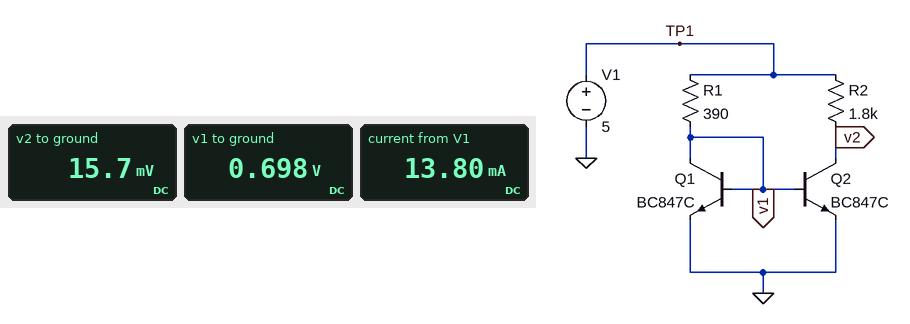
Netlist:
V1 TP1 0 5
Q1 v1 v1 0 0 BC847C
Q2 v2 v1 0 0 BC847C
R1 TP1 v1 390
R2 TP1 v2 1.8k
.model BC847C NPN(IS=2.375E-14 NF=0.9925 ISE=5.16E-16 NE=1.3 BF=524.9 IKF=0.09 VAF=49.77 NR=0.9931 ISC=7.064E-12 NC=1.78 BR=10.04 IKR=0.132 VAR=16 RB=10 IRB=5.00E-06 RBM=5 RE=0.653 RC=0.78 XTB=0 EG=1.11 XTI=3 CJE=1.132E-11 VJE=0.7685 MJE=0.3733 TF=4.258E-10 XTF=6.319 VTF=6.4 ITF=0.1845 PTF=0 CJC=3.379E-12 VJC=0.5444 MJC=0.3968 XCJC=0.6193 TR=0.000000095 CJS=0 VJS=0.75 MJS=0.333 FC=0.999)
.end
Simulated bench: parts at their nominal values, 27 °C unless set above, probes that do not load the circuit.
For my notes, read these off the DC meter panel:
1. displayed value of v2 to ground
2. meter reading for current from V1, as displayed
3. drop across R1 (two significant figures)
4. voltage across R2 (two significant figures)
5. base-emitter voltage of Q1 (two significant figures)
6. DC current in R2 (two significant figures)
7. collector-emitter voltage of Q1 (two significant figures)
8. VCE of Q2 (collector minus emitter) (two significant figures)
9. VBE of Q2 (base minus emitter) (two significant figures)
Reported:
15.7 mV
13.80 mA
4.3 V
5.0 V
700 mV
2.8 mA
700 mV
16 mV
700 mV
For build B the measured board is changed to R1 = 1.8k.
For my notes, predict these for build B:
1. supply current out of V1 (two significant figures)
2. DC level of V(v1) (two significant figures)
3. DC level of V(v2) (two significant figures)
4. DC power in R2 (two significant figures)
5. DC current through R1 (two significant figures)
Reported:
4.8 mA
650 mV
670 mV
10 mW
2.4 mA
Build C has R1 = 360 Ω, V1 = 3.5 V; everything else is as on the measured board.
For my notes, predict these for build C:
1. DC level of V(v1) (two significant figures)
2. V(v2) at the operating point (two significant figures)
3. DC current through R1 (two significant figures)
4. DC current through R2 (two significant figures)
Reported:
690 mV
14 mV
7.8 mA
1.9 mA
